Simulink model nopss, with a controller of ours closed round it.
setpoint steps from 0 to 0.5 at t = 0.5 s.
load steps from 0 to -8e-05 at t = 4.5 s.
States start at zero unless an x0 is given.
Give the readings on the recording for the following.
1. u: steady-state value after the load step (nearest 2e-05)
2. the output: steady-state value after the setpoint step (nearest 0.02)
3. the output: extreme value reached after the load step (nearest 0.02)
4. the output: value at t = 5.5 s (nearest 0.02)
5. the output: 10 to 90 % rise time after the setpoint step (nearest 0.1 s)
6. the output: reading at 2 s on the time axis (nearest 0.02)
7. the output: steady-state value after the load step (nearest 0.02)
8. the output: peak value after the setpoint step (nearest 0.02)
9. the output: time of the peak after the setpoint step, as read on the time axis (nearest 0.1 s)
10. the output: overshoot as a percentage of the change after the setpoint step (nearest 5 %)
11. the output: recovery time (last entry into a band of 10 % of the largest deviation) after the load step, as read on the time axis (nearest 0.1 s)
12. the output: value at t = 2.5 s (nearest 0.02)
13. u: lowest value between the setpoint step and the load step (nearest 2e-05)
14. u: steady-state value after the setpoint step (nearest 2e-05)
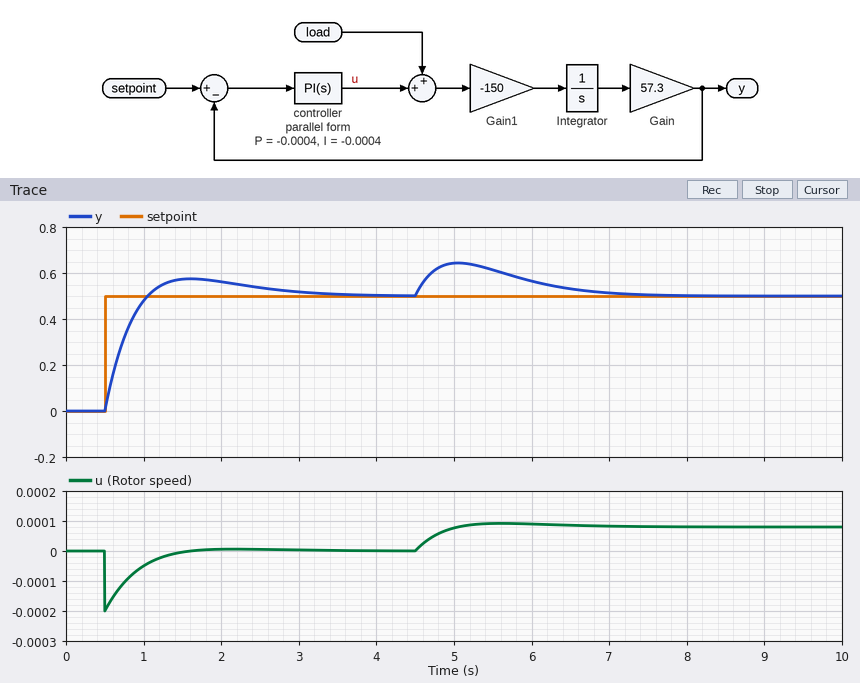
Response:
0.00008
0.50
0.64
0.62
0.4 s
0.56
0.50
0.58
1.6 s
15 %
7.0 s
0.54
-0.00020
0.00000
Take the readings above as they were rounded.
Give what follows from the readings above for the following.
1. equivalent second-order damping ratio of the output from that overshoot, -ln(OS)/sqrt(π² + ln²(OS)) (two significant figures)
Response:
0.52
